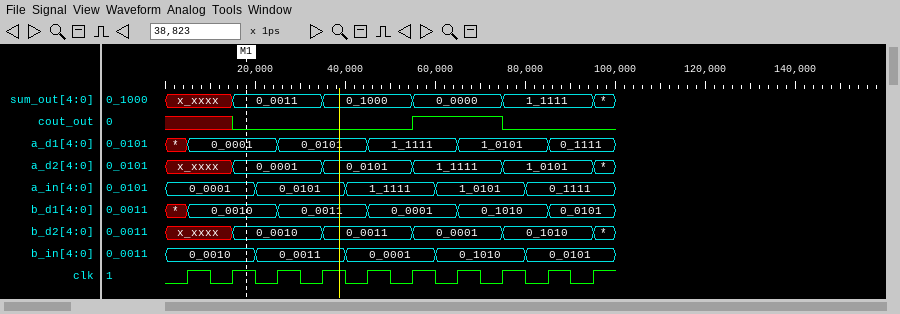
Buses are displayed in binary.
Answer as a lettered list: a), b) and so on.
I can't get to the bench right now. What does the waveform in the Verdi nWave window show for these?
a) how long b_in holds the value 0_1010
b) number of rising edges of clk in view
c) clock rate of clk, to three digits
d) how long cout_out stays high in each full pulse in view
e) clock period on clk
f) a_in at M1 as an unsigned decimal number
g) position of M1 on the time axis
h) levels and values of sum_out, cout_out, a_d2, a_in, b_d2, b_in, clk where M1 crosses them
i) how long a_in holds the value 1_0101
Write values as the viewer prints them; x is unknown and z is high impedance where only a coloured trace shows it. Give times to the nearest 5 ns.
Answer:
a) 20 ns
b) 10
c) 100 MHz
d) 20 ns
e) 10 ns
f) 1
g) 20 ns
h) sum_out=0_0011, cout_out=0, a_d2=0_0001, a_in=0_0001, b_d2=0_0010, b_in=0_0010, clk=1
i) 20 ns
